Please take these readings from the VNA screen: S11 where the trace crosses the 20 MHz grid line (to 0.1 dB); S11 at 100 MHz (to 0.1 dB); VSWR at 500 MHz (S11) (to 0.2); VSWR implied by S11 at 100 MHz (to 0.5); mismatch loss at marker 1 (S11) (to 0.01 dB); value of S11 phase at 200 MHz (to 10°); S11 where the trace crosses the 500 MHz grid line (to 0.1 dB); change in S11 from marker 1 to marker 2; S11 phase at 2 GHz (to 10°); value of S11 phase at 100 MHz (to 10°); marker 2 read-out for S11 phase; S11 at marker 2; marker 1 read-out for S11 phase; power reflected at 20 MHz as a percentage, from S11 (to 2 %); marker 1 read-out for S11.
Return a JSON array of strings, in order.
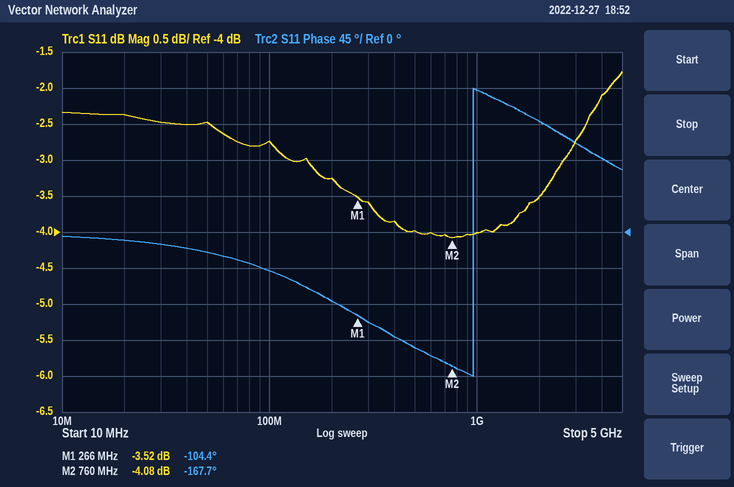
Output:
["-2.4 dB", "-2.7 dB", "4.4", "6.5", "2.55 dB", "-90°", "-4.0 dB", "-0.56 dB", "140°", "-50°", "-167.7°", "-4.08 dB", "-104.4°", "58 %", "-3.52 dB"]
